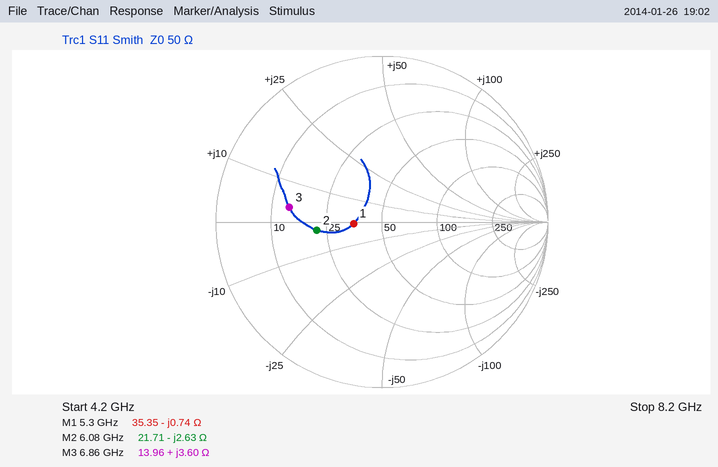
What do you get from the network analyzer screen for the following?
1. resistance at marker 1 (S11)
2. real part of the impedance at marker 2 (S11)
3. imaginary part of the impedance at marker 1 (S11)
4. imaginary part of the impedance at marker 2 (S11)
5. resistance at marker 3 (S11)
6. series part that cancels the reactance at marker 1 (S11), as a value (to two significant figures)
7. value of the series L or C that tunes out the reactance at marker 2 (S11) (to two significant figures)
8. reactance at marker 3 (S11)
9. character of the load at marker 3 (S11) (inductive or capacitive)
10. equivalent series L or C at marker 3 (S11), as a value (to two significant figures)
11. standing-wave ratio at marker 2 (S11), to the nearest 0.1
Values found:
35.35 Ω
21.71 Ω
-0.74 Ω
-2.63 Ω
13.96 Ω
22 pH
69 pH
+3.60 Ω
inductive
84 pH
2.3
